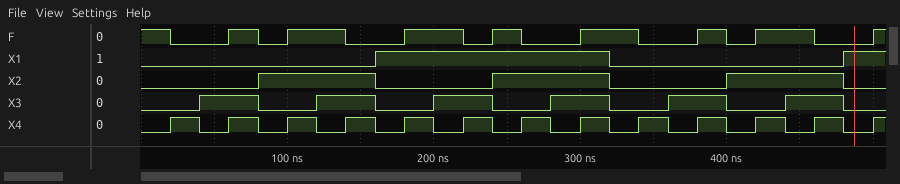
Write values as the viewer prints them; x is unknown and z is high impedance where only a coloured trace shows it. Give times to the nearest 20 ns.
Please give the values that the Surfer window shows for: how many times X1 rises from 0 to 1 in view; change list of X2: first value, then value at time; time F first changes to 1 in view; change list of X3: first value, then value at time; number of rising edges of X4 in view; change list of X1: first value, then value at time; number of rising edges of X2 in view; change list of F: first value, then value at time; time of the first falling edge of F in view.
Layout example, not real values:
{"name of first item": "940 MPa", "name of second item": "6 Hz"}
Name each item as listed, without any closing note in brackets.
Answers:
{"how many times X1 rises from 0 to 1 in view": "2", "change list of X2: first value, then value at time": "0, 1 at 80 ns, 0 at 160 ns, 1 at 240 ns, 0 at 320 ns, 1 at 400 ns, 0 at 480 ns", "time F first changes to 1 in view": "60 ns", "change list of X3: first value, then value at time": "0, 1 at 40 ns, 0 at 80 ns, 1 at 120 ns, 0 at 160 ns, 1 at 200 ns, 0 at 240 ns, 1 at 280 ns, 0 at 320 ns, 1 at 360 ns, 0 at 400 ns, 1 at 440 ns, 0 at 480 ns", "number of rising edges of X4 in view": "13", "change list of X1: first value, then value at time": "0, 1 at 160 ns, 0 at 320 ns, 1 at 480 ns", "number of rising edges of X2 in view": "3", "change list of F: first value, then value at time": "1, 0 at 20 ns, 1 at 60 ns, 0 at 80 ns, 1 at 100 ns, 0 at 140 ns, 1 at 180 ns, 0 at 220 ns, 1 at 240 ns, 0 at 260 ns, 1 at 300 ns, 0 at 340 ns, 1 at 380 ns, 0 at 400 ns, 1 at 420 ns, 0 at 460 ns, 1 at 500 ns", "time of the first falling edge of F in view": "20 ns"}
